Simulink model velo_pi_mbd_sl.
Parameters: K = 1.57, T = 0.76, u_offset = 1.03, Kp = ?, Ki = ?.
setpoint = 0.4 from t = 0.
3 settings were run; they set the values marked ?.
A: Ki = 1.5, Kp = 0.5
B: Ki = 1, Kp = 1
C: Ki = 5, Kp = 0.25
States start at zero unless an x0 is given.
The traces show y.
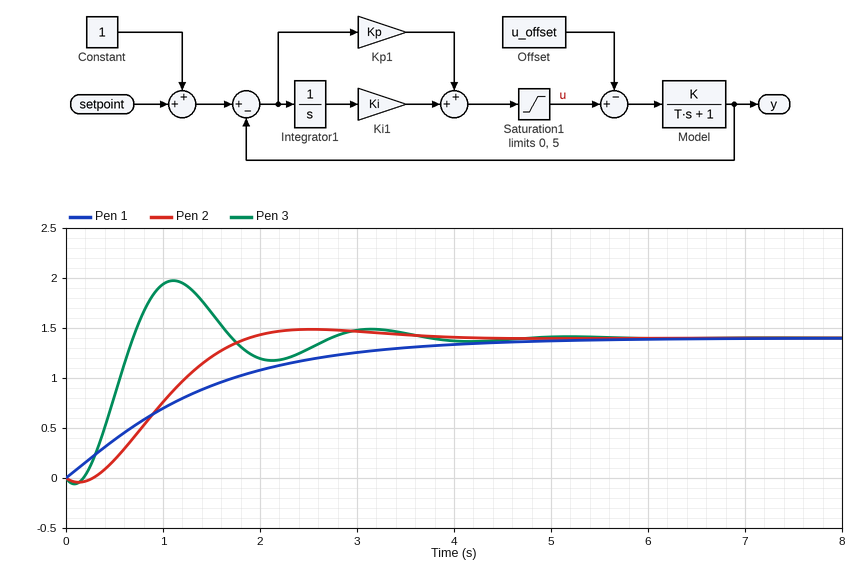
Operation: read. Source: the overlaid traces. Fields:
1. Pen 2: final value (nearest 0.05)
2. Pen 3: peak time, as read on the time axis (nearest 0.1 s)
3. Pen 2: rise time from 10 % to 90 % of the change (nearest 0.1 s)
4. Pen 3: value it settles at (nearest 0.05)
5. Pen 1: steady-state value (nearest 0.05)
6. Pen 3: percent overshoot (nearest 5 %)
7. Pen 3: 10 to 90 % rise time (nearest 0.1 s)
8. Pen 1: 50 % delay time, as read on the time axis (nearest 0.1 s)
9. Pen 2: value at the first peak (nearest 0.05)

1.40
1.1 s
1.1 s
1.40
1.40
40 %
0.4 s
1.0 s
1.50
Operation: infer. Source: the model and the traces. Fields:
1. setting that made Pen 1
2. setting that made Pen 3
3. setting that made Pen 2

B
C
A
